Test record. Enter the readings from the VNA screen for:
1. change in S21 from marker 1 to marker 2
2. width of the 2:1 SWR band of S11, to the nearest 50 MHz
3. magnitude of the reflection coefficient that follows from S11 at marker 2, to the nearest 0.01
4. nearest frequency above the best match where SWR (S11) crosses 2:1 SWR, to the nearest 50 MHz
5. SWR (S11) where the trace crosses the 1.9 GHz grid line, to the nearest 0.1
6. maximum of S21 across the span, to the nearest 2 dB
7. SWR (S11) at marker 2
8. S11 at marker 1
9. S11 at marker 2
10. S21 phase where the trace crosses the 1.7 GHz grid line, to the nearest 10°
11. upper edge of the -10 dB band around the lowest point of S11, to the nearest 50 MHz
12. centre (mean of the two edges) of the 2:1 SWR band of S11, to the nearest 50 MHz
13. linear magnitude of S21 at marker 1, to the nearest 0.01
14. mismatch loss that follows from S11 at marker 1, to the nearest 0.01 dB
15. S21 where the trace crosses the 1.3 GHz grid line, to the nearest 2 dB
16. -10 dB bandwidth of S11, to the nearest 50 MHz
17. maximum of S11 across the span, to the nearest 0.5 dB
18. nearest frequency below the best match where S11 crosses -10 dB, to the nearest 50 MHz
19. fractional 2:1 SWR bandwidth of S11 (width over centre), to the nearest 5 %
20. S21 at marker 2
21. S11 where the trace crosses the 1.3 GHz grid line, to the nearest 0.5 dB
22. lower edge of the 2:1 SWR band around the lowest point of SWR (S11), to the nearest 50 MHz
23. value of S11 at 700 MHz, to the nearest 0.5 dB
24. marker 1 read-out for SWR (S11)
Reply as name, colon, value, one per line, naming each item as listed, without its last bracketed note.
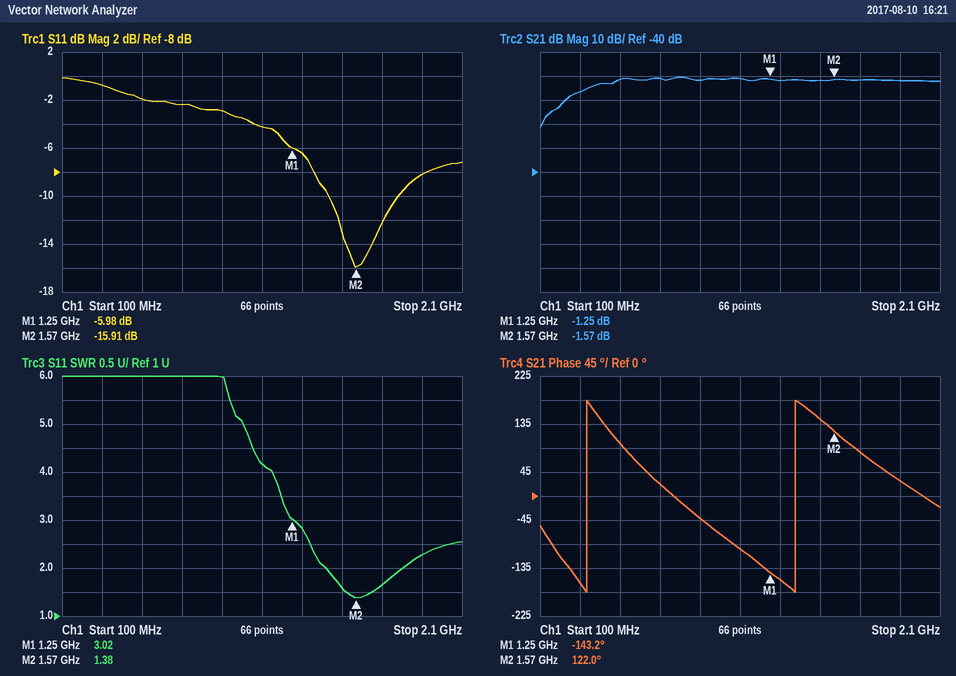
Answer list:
change in S21 from marker 1 to marker 2: -0.32 dB
width of the 2:1 SWR band of S11, to the nearest 50 MHz: 400 MHz
magnitude of the reflection coefficient that follows from S11 at marker 2, to the nearest 0.01: 0.16
nearest frequency above the best match where SWR (S11) crosses 2:1 SWR, to the nearest 50 MHz: 1.80 GHz
SWR (S11) where the trace crosses the 1.9 GHz grid line, to the nearest 0.1: 2.3
maximum of S21 across the span, to the nearest 2 dB: 0 dB
SWR (S11) at marker 2: 1.38
S11 at marker 1: -5.98 dB
S11 at marker 2: -15.91 dB
S21 phase where the trace crosses the 1.7 GHz grid line, to the nearest 10°: 80°
upper edge of the -10 dB band around the lowest point of S11, to the nearest 50 MHz: 1.80 GHz
centre (mean of the two edges) of the 2:1 SWR band of S11, to the nearest 50 MHz: 1.60 GHz
linear magnitude of S21 at marker 1, to the nearest 0.01: 0.87
mismatch loss that follows from S11 at marker 1, to the nearest 0.01 dB: 1.26 dB
S21 where the trace crosses the 1.3 GHz grid line, to the nearest 2 dB: -2 dB
-10 dB bandwidth of S11, to the nearest 50 MHz: 350 MHz
maximum of S11 across the span, to the nearest 0.5 dB: 0.0 dB
nearest frequency below the best match where S11 crosses -10 dB, to the nearest 50 MHz: 1.45 GHz
fractional 2:1 SWR bandwidth of S11 (width over centre), to the nearest 5 %: 25 %
S21 at marker 2: -1.57 dB
S11 where the trace crosses the 1.3 GHz grid line, to the nearest 0.5 dB: -6.5 dB
lower edge of the 2:1 SWR band around the lowest point of SWR (S11), to the nearest 50 MHz: 1.40 GHz
value of S11 at 700 MHz, to the nearest 0.5 dB: -2.5 dB
marker 1 read-out for SWR: 3.02
